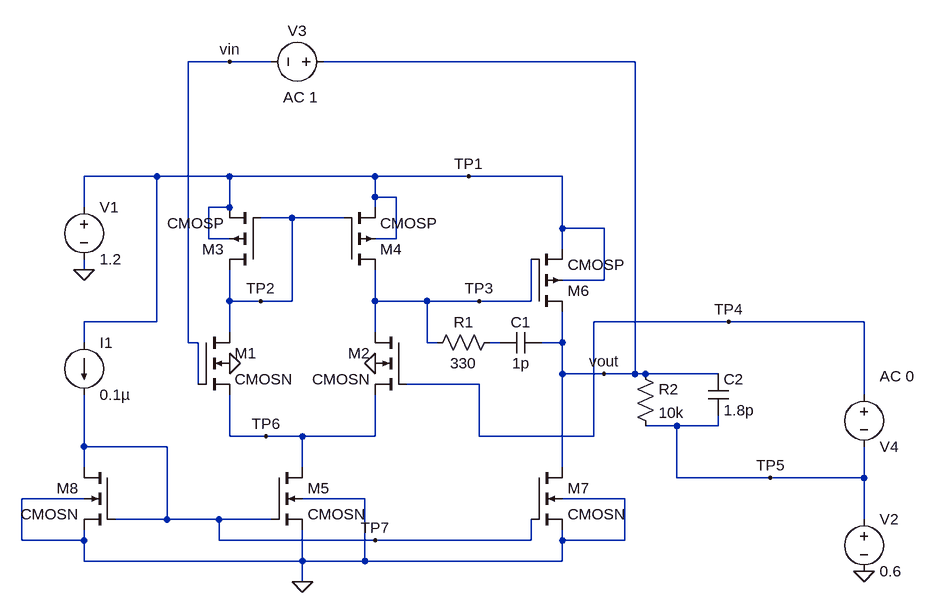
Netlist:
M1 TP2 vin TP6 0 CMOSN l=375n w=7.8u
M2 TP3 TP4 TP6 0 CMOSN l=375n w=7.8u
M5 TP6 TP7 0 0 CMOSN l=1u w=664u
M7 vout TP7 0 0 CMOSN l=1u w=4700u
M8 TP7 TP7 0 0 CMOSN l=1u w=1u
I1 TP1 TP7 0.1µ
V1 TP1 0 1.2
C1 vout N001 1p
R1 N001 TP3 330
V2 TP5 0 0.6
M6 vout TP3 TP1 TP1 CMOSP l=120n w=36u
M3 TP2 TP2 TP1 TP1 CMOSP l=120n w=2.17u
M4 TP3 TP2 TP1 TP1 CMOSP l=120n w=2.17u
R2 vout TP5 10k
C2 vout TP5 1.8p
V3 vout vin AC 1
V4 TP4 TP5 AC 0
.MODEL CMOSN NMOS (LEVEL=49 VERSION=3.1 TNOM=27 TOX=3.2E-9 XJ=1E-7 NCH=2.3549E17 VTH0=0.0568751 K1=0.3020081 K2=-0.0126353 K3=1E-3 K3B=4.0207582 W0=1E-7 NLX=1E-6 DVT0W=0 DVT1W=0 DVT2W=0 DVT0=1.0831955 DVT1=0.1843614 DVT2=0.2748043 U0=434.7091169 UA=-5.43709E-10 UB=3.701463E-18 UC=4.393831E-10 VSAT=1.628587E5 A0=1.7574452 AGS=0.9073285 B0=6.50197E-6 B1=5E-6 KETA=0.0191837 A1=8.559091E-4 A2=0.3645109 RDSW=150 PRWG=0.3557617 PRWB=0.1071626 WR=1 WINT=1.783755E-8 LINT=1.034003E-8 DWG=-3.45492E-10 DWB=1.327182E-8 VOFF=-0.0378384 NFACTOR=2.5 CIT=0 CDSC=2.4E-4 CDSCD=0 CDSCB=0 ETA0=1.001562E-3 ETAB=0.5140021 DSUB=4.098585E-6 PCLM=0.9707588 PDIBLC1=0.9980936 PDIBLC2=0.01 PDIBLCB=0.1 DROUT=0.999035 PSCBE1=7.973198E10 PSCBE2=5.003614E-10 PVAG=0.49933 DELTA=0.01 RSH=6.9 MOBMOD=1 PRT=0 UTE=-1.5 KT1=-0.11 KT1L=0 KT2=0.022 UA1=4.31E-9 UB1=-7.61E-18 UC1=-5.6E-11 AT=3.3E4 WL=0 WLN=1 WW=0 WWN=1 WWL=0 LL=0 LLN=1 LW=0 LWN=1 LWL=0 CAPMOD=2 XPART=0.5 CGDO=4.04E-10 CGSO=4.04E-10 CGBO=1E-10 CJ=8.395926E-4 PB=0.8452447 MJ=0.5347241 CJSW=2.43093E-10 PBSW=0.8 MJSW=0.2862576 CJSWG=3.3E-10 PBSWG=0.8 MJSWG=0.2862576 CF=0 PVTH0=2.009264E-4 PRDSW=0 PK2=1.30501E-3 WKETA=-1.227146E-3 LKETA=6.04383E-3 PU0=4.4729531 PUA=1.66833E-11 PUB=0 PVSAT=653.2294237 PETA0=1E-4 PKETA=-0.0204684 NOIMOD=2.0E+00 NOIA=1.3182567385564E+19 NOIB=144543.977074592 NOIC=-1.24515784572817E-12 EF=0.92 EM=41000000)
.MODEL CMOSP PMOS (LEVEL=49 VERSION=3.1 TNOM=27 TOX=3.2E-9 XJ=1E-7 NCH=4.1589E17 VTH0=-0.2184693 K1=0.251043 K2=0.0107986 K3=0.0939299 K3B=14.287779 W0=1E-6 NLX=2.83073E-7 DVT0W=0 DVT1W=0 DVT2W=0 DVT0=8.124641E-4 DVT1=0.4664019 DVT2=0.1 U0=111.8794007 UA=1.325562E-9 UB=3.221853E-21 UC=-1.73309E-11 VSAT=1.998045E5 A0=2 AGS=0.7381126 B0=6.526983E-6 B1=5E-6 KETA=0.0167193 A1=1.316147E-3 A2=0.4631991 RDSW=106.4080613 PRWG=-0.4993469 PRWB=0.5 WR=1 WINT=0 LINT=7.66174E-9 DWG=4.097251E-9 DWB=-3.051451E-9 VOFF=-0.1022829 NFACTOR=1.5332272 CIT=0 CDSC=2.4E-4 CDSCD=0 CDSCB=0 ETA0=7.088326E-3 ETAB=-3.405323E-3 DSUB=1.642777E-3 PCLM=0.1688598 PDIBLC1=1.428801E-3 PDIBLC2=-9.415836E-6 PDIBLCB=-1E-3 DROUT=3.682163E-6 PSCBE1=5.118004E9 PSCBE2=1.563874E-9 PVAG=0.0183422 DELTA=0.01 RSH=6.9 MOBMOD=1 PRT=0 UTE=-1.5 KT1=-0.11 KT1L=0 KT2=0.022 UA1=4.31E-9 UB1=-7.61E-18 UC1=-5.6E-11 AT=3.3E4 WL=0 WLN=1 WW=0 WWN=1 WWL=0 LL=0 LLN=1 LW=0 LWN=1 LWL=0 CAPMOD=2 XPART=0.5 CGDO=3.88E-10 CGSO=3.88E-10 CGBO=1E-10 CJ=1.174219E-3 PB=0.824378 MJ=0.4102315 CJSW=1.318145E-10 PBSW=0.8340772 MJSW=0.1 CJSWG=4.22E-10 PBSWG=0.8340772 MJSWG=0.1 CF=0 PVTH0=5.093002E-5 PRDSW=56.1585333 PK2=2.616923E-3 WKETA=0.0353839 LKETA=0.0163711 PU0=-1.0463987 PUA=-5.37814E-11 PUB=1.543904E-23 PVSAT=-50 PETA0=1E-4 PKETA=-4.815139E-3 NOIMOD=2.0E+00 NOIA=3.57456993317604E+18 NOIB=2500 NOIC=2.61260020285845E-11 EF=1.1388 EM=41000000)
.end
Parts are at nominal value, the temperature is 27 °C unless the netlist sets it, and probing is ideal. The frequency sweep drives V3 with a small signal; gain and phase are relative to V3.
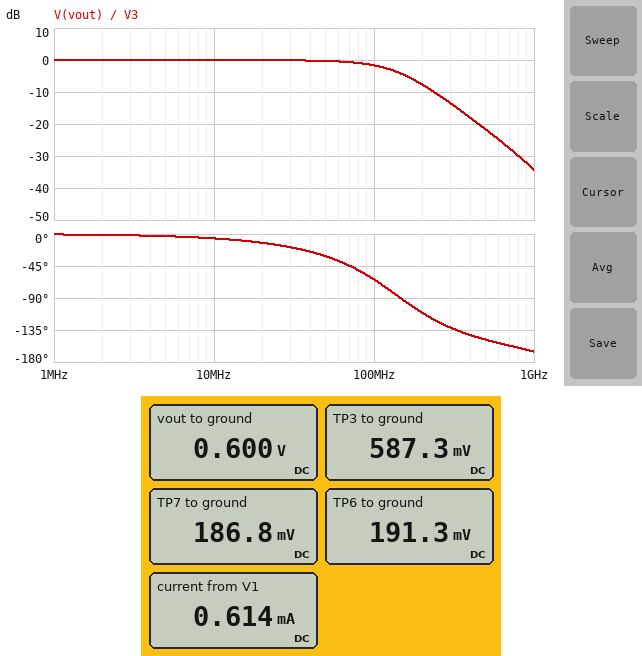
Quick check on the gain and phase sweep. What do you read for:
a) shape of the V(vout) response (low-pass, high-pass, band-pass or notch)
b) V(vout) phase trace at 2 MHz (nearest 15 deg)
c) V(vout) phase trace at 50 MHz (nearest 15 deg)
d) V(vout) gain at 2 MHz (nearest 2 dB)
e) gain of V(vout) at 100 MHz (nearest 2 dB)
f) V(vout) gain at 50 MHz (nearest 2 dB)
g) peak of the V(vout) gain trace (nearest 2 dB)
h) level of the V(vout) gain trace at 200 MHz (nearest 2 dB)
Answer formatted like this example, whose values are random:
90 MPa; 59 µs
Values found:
low-pass; 0 deg; -30 deg; 0 dB; -2 dB; 0 dB; 0 dB; -8 dB
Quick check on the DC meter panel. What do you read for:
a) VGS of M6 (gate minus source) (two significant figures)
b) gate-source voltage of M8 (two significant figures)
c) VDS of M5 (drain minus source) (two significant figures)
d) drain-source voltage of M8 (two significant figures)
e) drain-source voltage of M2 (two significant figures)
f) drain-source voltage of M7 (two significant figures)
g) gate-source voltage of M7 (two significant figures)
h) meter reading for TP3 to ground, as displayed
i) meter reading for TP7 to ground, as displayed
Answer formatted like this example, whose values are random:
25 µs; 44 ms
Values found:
-610 mV; 190 mV; 190 mV; 190 mV; 400 mV; 600 mV; 190 mV; 587.3 mV; 186.8 mV
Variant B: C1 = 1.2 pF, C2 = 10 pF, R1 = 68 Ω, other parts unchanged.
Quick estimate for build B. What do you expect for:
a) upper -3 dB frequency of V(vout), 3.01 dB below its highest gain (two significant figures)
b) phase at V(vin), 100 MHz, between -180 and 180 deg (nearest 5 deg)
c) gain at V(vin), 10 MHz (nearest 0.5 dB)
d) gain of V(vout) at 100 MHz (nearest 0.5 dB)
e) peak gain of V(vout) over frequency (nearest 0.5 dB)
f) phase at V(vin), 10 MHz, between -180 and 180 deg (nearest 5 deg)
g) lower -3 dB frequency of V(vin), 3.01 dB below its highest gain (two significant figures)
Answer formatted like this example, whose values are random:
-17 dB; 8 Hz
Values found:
89 MHz; -160 deg; -17.5 dB; -3.0 dB; 2.0 dB; -90 deg; 56 MHz
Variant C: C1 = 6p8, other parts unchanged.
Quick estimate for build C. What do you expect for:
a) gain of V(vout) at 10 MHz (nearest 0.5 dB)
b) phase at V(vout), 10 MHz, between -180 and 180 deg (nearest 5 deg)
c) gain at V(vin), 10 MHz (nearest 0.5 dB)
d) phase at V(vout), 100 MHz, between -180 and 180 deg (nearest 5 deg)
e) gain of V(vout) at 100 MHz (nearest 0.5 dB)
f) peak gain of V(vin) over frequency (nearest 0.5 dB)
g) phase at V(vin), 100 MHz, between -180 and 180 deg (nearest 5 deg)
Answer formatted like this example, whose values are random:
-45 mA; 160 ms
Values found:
-2.0 dB; -35 deg; -5.0 dB; -80 deg; -16.5 dB; 0 dB; -170 deg
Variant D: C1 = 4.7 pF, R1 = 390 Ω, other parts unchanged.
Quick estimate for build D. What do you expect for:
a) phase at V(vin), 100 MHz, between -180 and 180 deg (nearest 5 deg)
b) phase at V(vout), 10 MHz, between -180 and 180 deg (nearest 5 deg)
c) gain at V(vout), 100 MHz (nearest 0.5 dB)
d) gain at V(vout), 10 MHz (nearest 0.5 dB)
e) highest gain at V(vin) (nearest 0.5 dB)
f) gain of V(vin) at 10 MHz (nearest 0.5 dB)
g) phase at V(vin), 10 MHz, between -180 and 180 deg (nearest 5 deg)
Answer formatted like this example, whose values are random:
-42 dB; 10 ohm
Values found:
-170 deg; -25 deg; -13.5 dB; -1.0 dB; 0 dB; -7.0 dB; -115 deg
